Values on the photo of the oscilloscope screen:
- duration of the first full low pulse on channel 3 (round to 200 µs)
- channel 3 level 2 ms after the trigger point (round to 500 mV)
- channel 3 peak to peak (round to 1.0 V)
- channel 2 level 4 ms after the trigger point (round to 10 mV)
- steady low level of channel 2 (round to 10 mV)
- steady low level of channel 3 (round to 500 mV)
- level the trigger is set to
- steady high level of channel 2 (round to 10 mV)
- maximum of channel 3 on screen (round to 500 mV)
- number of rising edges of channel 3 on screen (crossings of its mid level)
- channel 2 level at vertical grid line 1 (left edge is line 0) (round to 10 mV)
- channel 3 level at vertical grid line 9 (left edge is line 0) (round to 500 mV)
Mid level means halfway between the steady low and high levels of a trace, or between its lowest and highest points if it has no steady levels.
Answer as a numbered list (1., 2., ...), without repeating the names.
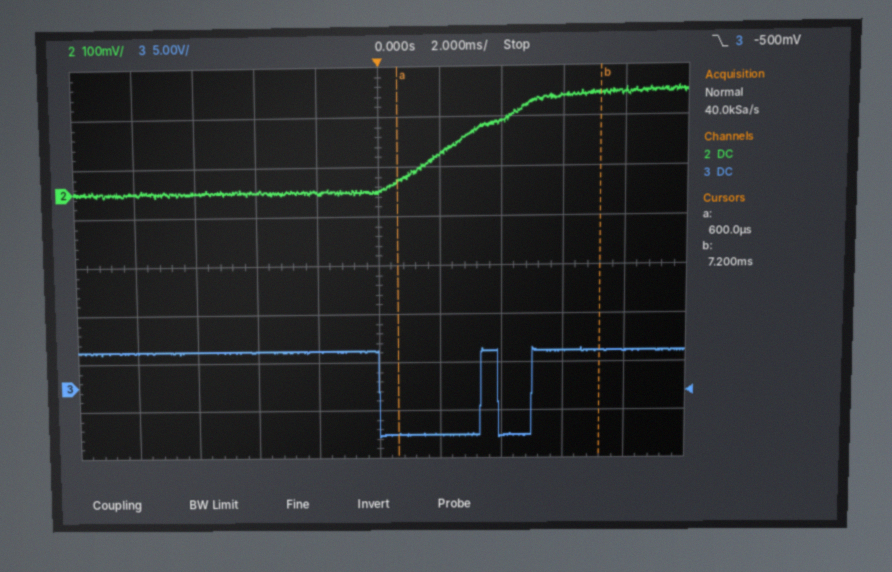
1. 3.4 ms
2. -5.0 V
3. 9.0 V
4. 140 mV
5. 0 mV
6. -5.0 V
7. -500 mV
8. 200 mV
9. 4.0 V
10. 2
11. 0 mV
12. 3.5 V
